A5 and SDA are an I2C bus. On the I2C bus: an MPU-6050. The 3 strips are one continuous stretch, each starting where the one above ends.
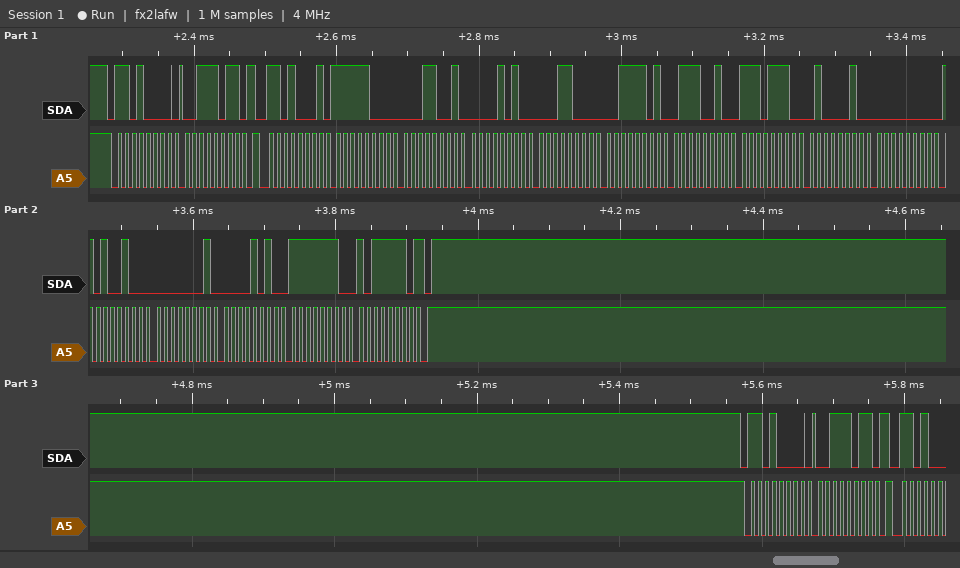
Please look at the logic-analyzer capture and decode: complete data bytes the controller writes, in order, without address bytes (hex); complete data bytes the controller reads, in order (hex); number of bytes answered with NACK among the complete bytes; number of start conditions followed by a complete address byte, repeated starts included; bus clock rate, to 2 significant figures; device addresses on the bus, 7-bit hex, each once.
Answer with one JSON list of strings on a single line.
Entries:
["3B 3B", "F8 19 0A 18 3D 72 EE 42 00 A4 01 0A FE BE", "1", "3", "100 kHz", "0x68"]
